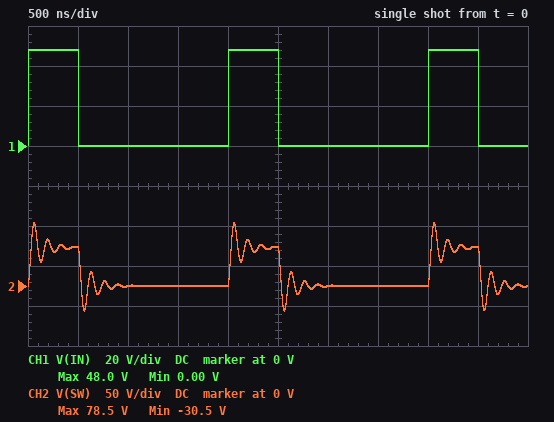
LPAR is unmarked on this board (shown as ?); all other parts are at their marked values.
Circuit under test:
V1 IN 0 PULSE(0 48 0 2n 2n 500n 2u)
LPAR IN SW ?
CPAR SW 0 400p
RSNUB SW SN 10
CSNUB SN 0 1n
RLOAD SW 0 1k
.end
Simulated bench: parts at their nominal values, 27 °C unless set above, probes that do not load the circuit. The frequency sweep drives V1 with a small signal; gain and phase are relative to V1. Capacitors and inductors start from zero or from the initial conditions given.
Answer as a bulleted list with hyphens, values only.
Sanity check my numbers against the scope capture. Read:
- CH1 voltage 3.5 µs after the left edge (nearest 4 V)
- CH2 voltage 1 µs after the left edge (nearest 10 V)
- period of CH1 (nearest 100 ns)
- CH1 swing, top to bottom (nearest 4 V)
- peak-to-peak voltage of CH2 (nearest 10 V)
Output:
- 0 V
- 0 V
- 2.0 µs
- 48 V
- 110 V
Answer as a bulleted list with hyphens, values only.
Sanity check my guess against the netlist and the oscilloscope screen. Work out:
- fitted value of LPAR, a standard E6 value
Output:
- 330 nH
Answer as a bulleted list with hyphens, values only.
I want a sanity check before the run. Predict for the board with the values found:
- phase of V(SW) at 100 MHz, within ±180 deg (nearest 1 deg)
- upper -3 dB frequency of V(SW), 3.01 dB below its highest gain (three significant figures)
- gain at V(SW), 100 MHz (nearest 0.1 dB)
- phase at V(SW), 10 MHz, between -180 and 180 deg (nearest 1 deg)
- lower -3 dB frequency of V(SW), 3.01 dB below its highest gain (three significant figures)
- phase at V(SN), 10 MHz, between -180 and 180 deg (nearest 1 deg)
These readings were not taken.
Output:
- -159 deg
- 8.63 MHz
- -35.3 dB
- -127 deg
- 5.93 MHz
- -159 deg
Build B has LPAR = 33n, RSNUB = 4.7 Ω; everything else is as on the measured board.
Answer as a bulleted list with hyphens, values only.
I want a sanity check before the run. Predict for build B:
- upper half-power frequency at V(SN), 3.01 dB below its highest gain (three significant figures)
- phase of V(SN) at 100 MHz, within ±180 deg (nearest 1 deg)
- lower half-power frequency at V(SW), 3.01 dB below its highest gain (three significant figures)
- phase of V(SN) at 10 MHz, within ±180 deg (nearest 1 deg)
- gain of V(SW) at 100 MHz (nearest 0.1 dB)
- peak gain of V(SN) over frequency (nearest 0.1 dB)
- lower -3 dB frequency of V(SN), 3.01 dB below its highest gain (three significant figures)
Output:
- 28.7 MHz
- 144 deg
- 16.7 MHz
- -19 deg
- -16.7 dB
- 6.1 dB
- 15.1 MHz
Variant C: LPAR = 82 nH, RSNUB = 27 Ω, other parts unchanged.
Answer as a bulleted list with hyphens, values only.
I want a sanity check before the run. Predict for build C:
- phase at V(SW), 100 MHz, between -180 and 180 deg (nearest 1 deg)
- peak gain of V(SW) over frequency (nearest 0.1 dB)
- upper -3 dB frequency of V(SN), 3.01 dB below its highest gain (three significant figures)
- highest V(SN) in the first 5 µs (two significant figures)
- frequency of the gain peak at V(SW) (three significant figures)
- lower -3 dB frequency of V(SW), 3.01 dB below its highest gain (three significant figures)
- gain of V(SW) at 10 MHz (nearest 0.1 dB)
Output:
- -171 deg
- 6.6 dB
- 7.74 MHz
- 48 V
- 24.0 MHz
- 15.0 MHz
- 1.9 dB
